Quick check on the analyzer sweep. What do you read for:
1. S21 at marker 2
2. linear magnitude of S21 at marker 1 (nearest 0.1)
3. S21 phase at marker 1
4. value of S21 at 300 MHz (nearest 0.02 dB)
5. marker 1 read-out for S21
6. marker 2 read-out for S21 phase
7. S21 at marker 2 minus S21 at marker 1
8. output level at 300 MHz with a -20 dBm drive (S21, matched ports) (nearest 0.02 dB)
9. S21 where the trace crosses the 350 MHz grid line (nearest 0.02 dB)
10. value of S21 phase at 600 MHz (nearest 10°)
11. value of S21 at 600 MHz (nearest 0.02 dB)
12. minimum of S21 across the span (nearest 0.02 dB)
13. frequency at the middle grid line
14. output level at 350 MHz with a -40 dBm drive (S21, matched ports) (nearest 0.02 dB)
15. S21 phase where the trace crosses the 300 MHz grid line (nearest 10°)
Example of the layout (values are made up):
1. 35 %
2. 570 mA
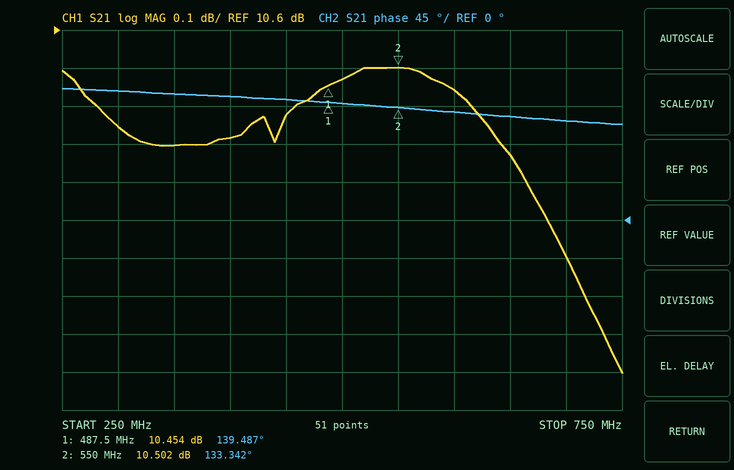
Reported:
1. 10.502 dB
2. 3.3
3. 139.487°
4. 10.34 dB
5. 10.454 dB
6. 133.342°
7. 0.048 dB
8. -9.66 dBm
9. 10.30 dB
10. 130°
11. 10.44 dB
12. 9.70 dB
13. 500 MHz
14. -29.70 dBm
15. 150°
